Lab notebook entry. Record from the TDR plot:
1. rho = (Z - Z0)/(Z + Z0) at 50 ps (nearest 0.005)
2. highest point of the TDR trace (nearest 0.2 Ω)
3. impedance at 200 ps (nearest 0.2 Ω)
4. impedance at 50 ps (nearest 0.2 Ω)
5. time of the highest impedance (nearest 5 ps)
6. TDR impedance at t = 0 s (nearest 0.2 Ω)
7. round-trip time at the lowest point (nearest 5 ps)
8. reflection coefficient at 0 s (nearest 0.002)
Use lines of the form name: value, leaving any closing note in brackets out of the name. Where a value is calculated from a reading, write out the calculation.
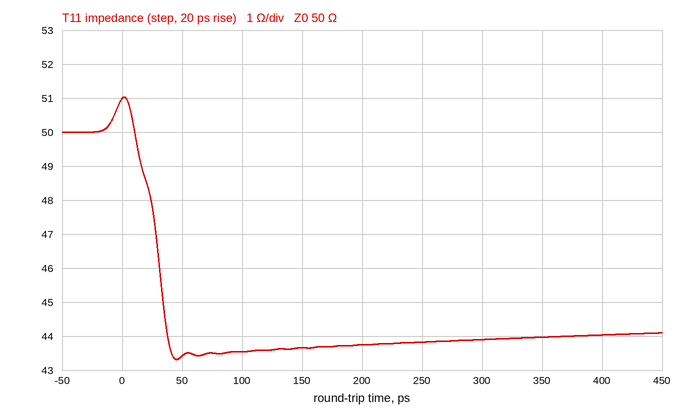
rho = (Z - Z0)/(Z + Z0) at 50 ps: (43.4 − 50)/(43.4 + 50) ≈ -0.0707, so -0.070 to the nearest 0.005
highest point of the TDR trace: 51.0 Ω
impedance at 200 ps: 43.8 Ω
impedance at 50 ps: 43.4 Ω
time of the highest impedance: 0 ps
TDR impedance at t = 0 s: 51.0 Ω
round-trip time at the lowest point: 45 ps
reflection coefficient at 0 s: (51 − 50)/(51 + 50) ≈ +0.010
